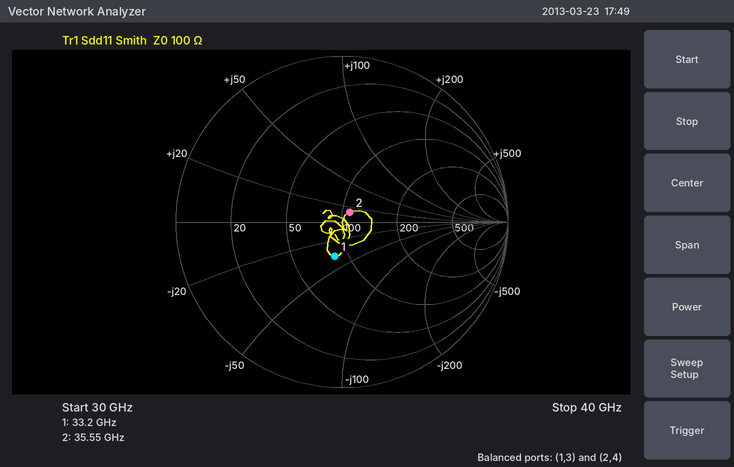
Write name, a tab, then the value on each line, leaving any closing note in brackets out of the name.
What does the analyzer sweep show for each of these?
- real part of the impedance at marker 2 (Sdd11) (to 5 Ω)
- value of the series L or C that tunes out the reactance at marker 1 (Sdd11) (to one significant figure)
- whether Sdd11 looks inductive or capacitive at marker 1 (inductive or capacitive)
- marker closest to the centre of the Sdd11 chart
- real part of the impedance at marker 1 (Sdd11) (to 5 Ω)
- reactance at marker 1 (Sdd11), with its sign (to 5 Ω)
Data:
real part of the impedance at marker 2 (Sdd11)	110 Ω
value of the series L or C that tunes out the reactance at marker 1 (Sdd11)	200 pH
whether Sdd11 looks inductive or capacitive at marker 1	capacitive
marker closest to the centre of the Sdd11 chart	marker 2
real part of the impedance at marker 1 (Sdd11)	85 Ω
reactance at marker 1 (Sdd11), with its sign	-35 Ω
